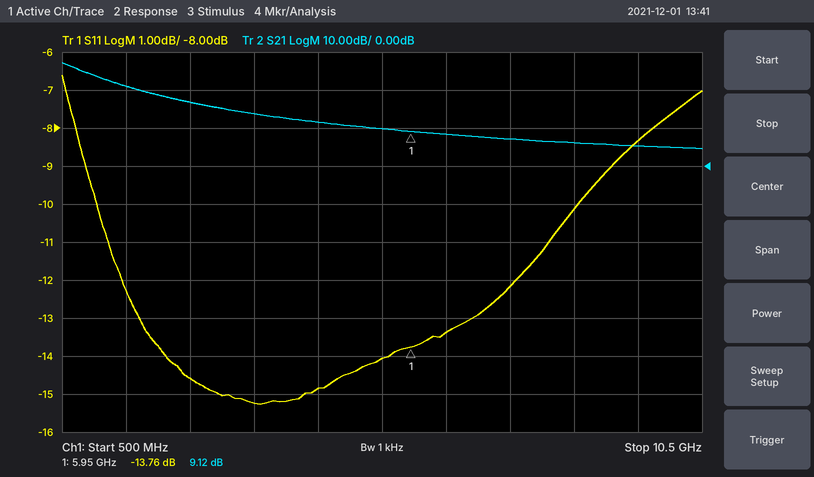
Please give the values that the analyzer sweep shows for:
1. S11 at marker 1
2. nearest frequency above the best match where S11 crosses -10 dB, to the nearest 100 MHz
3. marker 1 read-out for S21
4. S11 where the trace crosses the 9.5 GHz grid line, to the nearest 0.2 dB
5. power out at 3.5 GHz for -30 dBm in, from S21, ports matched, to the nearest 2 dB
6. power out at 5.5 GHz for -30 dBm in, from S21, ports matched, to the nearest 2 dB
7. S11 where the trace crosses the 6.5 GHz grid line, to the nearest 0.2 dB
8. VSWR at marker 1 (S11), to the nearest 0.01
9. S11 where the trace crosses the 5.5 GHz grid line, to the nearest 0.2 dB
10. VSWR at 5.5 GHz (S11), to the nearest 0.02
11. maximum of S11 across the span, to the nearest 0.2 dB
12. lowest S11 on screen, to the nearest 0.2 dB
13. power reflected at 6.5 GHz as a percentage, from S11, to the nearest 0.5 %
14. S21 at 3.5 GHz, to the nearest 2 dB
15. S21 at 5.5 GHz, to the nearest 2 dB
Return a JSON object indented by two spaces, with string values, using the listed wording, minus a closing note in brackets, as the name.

{
  "S11 at marker 1": "-13.76 dB",
  "nearest frequency above the best match where S11 crosses -10 dB, to the nearest 100 MHz": "8.6 GHz",
  "marker 1 read-out for S21": "9.12 dB",
  "S11 where the trace crosses the 9.5 GHz grid line, to the nearest 0.2 dB": "-8.4 dB",
  "power out at 3.5 GHz for -30 dBm in, from S21, ports matched, to the nearest 2 dB": "-16 dBm",
  "power out at 5.5 GHz for -30 dBm in, from S21, ports matched, to the nearest 2 dB": "-20 dBm",
  "S11 where the trace crosses the 6.5 GHz grid line, to the nearest 0.2 dB": "-13.4 dB",
  "VSWR at marker 1 (S11), to the nearest 0.01": "1.52",
  "S11 where the trace crosses the 5.5 GHz grid line, to the nearest 0.2 dB": "-14.0 dB",
  "VSWR at 5.5 GHz (S11), to the nearest 0.02": "1.50",
  "maximum of S11 across the span, to the nearest 0.2 dB": "-6.6 dB",
  "lowest S11 on screen, to the nearest 0.2 dB": "-15.2 dB",
  "power reflected at 6.5 GHz as a percentage, from S11, to the nearest 0.5 %": "4.5 %",
  "S21 at 3.5 GHz, to the nearest 2 dB": "14 dB",
  "S21 at 5.5 GHz, to the nearest 2 dB": "10 dB"
}
